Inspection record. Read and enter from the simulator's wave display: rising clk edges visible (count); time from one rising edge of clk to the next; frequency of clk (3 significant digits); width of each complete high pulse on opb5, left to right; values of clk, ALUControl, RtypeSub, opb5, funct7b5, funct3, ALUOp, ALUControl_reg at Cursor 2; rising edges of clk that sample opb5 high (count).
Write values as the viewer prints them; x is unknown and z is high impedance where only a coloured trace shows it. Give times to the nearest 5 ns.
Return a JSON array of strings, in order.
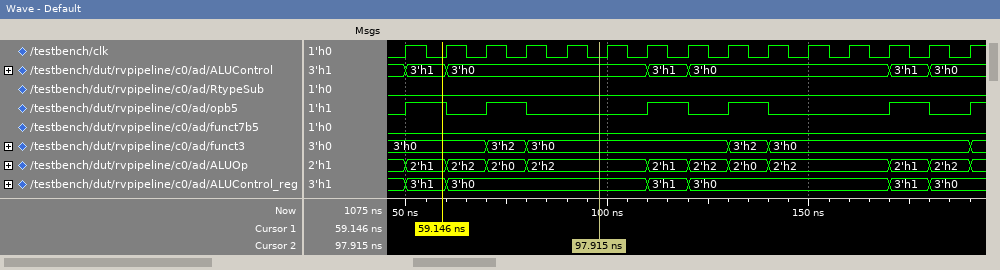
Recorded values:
["15", "10 ns", "100 MHz", "10 ns, 10 ns, 10 ns, 10 ns, 10 ns", "clk=0, ALUControl=3'h0, RtypeSub=0, opb5=0, funct7b5=0, funct3=3'h0, ALUOp=2'h2, ALUControl_reg=3'h0", "5"]
